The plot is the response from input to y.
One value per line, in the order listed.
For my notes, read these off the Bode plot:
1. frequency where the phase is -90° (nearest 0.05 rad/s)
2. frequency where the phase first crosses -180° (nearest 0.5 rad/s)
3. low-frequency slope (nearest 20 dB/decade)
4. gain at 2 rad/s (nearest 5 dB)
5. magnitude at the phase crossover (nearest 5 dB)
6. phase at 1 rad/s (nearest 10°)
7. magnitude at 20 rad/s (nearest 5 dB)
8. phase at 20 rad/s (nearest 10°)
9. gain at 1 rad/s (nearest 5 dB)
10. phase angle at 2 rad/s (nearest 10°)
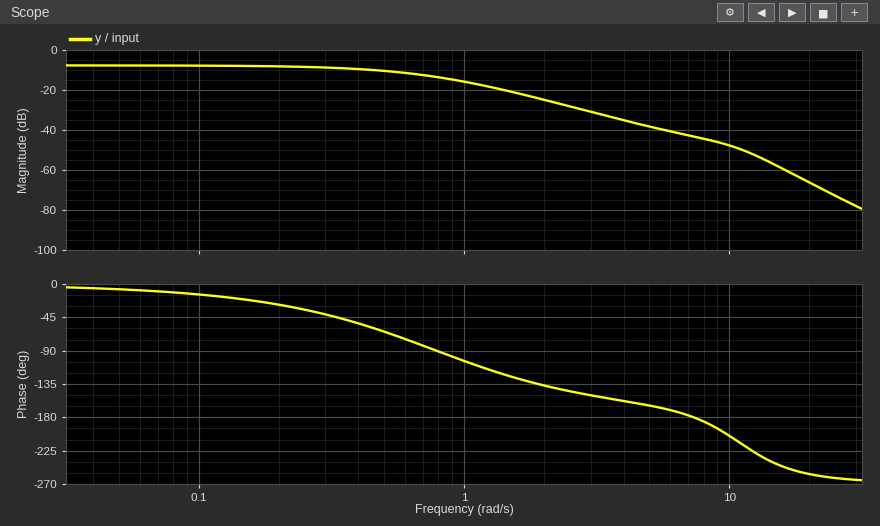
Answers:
0.80 rad/s
7.5 rad/s
0 dB/decade
-25 dB
-45 dB
-100°
-65 dB
-260°
-15 dB
-140°
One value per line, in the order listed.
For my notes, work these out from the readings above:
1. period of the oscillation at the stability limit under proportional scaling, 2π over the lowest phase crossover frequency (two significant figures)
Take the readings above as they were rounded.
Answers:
0.84 s
